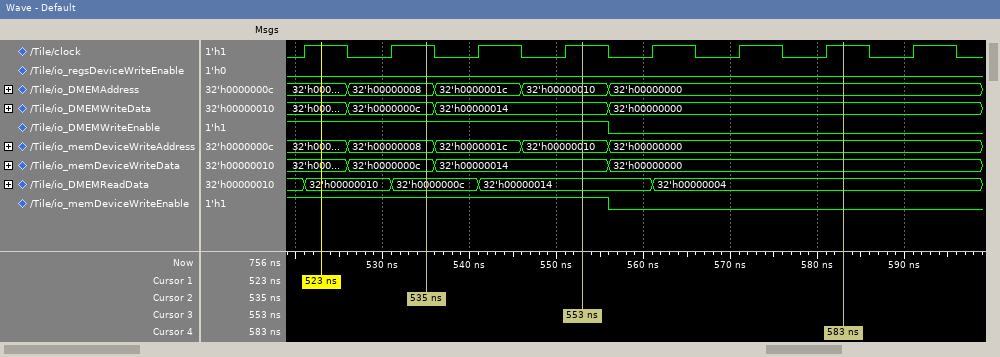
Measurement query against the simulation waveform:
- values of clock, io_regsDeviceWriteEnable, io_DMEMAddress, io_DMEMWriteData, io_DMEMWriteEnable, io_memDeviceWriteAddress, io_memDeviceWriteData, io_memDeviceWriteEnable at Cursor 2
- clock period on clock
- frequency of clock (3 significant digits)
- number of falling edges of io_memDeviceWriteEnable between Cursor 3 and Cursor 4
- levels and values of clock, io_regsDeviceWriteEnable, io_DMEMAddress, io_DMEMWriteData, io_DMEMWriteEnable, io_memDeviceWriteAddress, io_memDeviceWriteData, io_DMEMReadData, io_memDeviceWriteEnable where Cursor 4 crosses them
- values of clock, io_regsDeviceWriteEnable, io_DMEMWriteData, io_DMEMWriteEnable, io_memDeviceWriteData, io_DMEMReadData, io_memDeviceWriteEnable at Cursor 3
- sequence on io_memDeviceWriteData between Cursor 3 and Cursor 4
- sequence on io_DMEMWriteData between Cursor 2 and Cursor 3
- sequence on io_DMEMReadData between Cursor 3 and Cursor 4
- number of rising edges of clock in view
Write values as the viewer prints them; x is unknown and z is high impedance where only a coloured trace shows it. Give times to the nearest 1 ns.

clock=1, io_regsDeviceWriteEnable=0, io_DMEMAddress=32'h00000008, io_DMEMWriteData=32'h0000000c, io_DMEMWriteEnable=1, io_memDeviceWriteAddress=32'h00000008, io_memDeviceWriteData=32'h0000000c, io_memDeviceWriteEnable=1
10 ns
100 MHz
1
clock=1, io_regsDeviceWriteEnable=0, io_DMEMAddress=32'h00000000, io_DMEMWriteData=32'h00000000, io_DMEMWriteEnable=0, io_memDeviceWriteAddress=32'h00000000, io_memDeviceWriteData=32'h00000000, io_DMEMReadData=32'h00000004, io_memDeviceWriteEnable=0
clock=1, io_regsDeviceWriteEnable=0, io_DMEMWriteData=32'h00000014, io_DMEMWriteEnable=1, io_memDeviceWriteData=32'h00000014, io_DMEMReadData=32'h00000014, io_memDeviceWriteEnable=1
32'h00000014, 32'h00000000
32'h0000000c, 32'h00000014
32'h00000014, 32'h00000004
8
